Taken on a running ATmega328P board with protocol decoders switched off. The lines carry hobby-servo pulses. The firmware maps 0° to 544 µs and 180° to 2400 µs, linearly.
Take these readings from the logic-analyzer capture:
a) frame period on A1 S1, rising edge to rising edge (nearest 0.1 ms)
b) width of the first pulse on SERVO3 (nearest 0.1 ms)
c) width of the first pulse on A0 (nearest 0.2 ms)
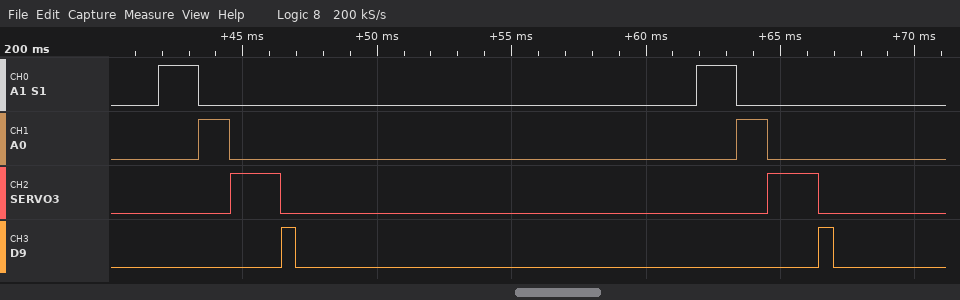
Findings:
20.0 ms
1.9 ms
1.2 ms
